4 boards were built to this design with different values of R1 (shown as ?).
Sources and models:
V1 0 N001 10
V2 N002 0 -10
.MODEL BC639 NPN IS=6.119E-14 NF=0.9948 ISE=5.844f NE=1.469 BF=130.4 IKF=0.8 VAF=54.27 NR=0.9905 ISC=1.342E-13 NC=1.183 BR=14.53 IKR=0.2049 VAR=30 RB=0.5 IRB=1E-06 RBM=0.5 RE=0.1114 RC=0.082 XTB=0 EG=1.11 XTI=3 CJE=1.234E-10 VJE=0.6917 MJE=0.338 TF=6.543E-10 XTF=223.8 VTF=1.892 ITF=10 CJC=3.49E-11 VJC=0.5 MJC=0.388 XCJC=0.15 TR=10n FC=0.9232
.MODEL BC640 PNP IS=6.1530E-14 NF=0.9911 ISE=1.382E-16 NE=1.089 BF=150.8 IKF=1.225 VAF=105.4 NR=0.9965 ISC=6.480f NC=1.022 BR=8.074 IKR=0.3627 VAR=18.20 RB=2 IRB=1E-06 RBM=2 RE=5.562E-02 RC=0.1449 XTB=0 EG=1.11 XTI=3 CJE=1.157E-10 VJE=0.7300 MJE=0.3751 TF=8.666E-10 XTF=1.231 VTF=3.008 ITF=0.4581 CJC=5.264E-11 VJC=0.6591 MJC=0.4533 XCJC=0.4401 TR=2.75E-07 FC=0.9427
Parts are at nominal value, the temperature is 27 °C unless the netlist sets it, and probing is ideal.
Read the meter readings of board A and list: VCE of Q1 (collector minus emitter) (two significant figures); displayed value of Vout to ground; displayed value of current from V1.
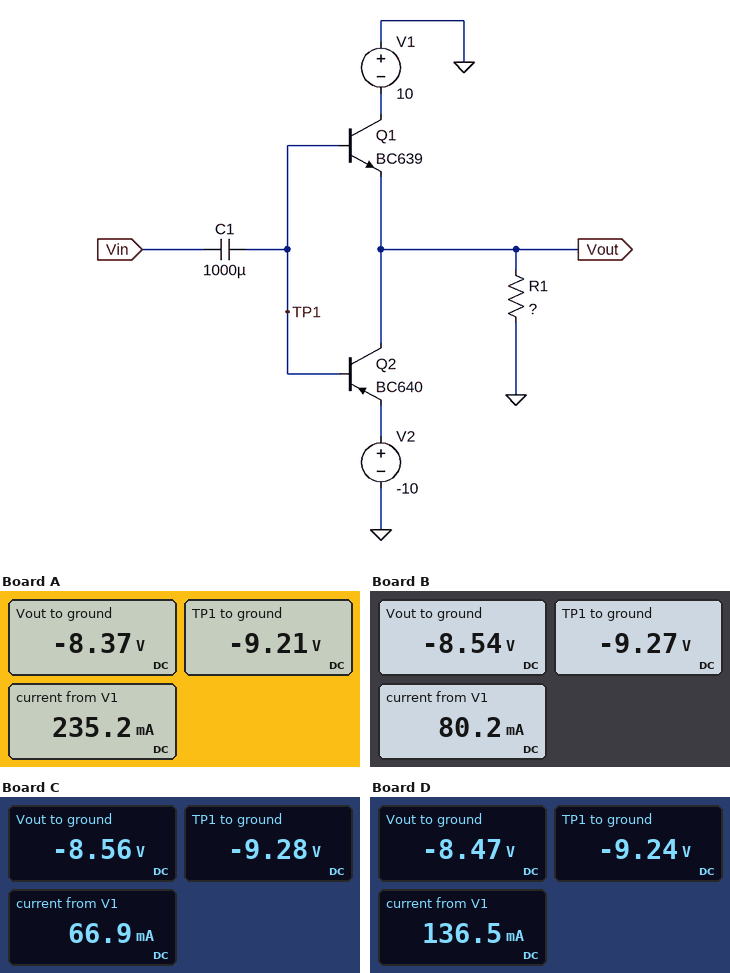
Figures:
-1.6 V
-8.37 V
235.2 mA
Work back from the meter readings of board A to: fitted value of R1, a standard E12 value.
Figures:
22 Ω
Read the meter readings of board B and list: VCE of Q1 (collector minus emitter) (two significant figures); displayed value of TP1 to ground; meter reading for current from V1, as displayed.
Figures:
-1.5 V
-9.27 V
80.2 mA
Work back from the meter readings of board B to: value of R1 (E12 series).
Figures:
68 Ω
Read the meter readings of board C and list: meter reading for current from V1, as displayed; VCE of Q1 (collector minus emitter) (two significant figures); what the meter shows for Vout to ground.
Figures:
66.9 mA
-1.4 V
-8.56 V
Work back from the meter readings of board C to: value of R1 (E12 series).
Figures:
82 Ω
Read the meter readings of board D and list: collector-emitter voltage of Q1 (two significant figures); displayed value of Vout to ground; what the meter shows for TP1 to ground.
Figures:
-1.5 V
-8.47 V
-9.24 V
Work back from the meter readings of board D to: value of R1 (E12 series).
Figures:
39 Ω
